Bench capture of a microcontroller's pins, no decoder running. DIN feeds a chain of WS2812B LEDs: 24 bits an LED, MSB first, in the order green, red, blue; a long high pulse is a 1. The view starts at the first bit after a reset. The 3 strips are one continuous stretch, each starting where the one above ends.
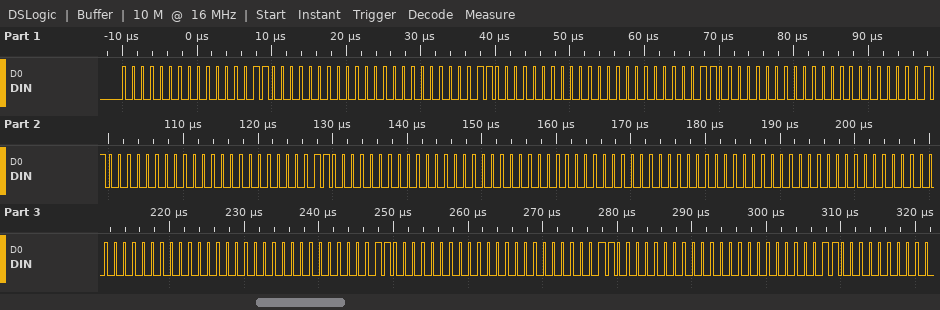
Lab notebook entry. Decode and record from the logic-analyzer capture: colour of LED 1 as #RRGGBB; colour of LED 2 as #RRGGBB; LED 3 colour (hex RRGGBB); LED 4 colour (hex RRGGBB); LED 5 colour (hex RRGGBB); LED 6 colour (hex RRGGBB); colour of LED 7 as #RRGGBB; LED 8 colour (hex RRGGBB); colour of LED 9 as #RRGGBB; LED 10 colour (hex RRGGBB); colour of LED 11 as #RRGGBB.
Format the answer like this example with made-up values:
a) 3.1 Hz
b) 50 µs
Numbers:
a) #030000
b) #030000
c) #030000
d) #030000
e) #030000
f) #000000
g) #000000
h) #000000
i) #030000
j) #030000
k) #030000
